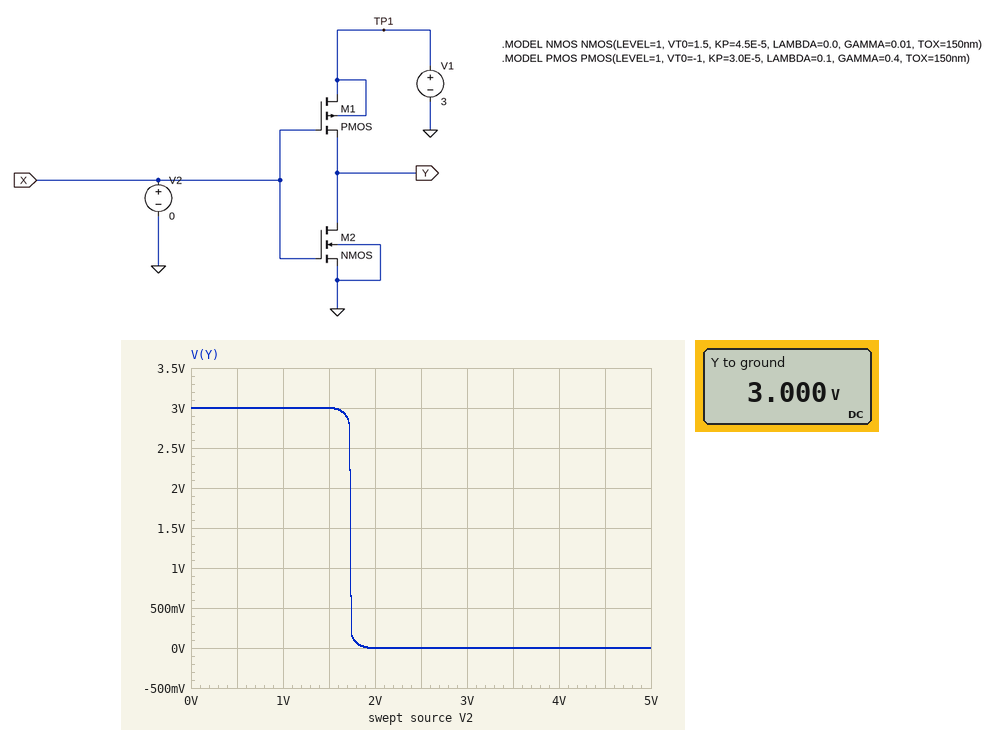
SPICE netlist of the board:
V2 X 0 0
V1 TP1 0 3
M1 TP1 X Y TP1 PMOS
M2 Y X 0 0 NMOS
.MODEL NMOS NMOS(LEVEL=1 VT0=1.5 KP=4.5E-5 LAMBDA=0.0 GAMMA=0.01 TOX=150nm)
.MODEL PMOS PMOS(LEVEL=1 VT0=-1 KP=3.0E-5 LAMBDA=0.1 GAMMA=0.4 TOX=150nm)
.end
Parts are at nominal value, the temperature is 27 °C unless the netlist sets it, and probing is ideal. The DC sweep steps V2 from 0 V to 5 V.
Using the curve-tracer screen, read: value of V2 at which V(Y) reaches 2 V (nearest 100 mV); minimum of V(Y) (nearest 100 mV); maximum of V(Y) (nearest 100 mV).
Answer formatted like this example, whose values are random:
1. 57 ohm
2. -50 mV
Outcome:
1. 1.7 V
2. 0 V
3. 3.0 V
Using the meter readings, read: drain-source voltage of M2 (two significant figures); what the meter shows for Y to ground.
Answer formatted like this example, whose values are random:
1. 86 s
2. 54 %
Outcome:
1. 3.0 V
2. 3.000 V
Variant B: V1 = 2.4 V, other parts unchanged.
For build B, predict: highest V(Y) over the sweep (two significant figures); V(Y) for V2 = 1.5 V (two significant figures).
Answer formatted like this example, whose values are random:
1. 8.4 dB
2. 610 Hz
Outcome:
1. 2.4 V
2. 1.2 V
